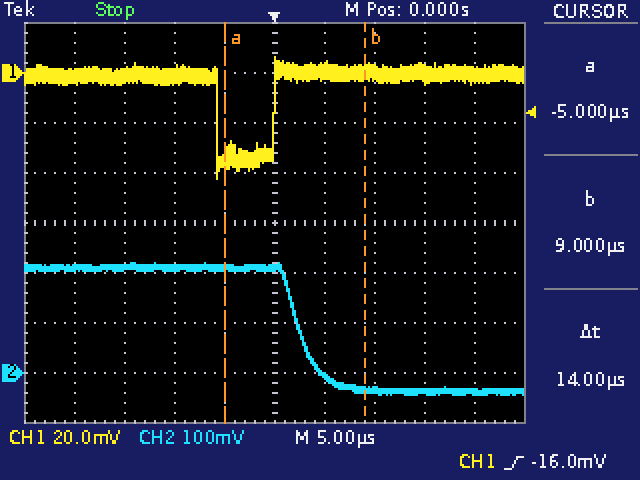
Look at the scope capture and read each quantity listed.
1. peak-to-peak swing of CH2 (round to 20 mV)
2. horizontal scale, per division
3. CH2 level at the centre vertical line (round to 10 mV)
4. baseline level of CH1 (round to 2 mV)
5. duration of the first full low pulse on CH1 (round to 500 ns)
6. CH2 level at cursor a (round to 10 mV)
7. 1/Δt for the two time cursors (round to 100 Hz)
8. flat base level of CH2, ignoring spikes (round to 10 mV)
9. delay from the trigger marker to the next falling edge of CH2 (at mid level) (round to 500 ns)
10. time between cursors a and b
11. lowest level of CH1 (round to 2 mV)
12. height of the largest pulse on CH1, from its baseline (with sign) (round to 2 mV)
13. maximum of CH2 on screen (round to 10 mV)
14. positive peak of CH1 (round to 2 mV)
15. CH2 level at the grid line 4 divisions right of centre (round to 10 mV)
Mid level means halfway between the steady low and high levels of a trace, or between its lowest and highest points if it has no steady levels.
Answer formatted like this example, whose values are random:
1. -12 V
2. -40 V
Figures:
1. 260 mV
2. 5 µs
3. 210 mV
4. 0 mV
5. 5.5 µs
6. 210 mV
7. 71.4 kHz
8. -40 mV
9. 2.5 µs
10. 14 µs
11. -42 mV
12. -42 mV
13. 220 mV
14. 6 mV
15. -40 mV
